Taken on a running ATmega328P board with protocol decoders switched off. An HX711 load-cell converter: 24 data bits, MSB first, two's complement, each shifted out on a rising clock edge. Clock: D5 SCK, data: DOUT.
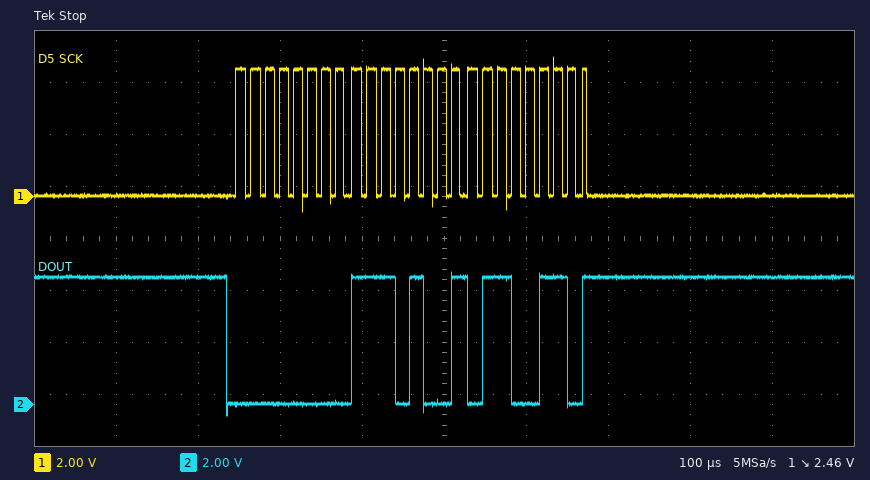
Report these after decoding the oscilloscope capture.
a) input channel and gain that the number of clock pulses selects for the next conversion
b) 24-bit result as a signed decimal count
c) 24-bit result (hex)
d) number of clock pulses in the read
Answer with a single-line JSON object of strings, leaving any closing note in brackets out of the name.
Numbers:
{"input channel and gain that the number of clock pulses selects for the next conversion": "channel A, gain 128", "24-bit result as a signed decimal count": "59750", "24-bit result": "0x00E966", "number of clock pulses in the read": "25"}
